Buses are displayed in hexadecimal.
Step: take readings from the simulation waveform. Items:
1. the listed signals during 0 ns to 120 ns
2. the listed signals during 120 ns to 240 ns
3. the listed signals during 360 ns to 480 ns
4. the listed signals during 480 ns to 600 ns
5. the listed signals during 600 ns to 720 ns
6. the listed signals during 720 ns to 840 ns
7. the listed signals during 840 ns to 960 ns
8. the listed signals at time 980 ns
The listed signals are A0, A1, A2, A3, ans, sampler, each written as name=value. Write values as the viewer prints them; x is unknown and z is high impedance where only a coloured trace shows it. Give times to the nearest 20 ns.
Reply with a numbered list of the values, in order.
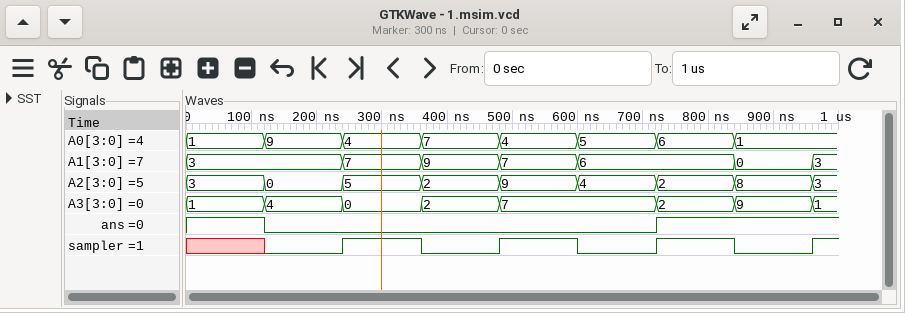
1. A0=1, A1=3, A2=3, A3=1, ans=1, sampler=x
2. A0=9, A1=3, A2=0, A3=4, ans=0, sampler=0
3. A0=7, A1=9, A2=2, A3=2, ans=0, sampler=0
4. A0=4, A1=7, A2=9, A3=7, ans=0, sampler=1
5. A0=5, A1=6, A2=4, A3=7, ans=0, sampler=0
6. A0=6, A1=6, A2=2, A3=2, ans=1, sampler=1
7. A0=1, A1=0, A2=8, A3=9, ans=1, sampler=0
8. A0=1, A1=3, A2=3, A3=1, ans=1, sampler=1
